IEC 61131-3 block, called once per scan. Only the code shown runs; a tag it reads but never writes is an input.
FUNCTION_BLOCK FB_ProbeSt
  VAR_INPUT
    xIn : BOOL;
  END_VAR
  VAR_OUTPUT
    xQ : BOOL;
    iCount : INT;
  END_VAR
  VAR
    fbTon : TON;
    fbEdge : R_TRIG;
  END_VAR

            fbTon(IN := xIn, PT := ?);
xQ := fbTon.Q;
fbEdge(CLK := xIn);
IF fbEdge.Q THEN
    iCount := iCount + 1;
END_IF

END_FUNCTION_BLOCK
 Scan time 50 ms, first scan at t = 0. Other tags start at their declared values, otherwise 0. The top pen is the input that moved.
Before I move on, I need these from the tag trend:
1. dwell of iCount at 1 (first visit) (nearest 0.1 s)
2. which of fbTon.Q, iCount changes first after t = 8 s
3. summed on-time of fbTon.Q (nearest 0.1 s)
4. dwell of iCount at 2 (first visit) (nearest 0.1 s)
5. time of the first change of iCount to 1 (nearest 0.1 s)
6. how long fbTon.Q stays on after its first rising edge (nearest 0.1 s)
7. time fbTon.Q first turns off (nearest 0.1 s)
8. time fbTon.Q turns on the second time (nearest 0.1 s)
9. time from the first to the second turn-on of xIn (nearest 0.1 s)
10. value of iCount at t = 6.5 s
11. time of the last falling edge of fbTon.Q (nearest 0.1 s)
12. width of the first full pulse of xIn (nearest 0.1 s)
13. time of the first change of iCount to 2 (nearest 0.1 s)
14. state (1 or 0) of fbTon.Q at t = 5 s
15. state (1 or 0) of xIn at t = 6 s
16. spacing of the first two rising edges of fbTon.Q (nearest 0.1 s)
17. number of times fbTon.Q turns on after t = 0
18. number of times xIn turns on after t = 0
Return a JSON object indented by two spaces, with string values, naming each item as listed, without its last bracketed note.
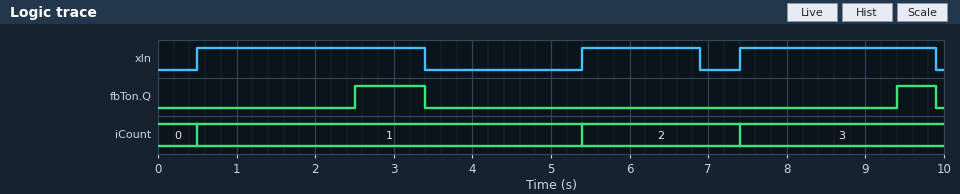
{
  "dwell of iCount at 1 (first visit)": "4.9 s",
  "which of fbTon.Q, iCount changes first after t = 8 s": "fbTon.Q",
  "summed on-time of fbTon.Q": "1.4 s",
  "dwell of iCount at 2 (first visit)": "2.0 s",
  "time of the first change of iCount to 1": "0.5 s",
  "how long fbTon.Q stays on after its first rising edge": "0.9 s",
  "time fbTon.Q first turns off": "3.4 s",
  "time fbTon.Q turns on the second time": "9.4 s",
  "time from the first to the second turn-on of xIn": "4.9 s",
  "value of iCount at t = 6.5 s": "2",
  "time of the last falling edge of fbTon.Q": "9.9 s",
  "width of the first full pulse of xIn": "2.9 s",
  "time of the first change of iCount to 2": "5.4 s",
  "state (1 or 0) of fbTon.Q at t = 5 s": "0",
  "state (1 or 0) of xIn at t = 6 s": "1",
  "spacing of the first two rising edges of fbTon.Q": "6.9 s",
  "number of times fbTon.Q turns on after t = 0": "2",
  "number of times xIn turns on after t = 0": "3"
}
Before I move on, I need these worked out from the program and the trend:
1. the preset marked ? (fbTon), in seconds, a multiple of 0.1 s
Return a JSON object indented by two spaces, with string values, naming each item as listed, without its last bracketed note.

{
  "the preset marked ? (fbTon), in seconds, a multiple of 0.1 s": "2.0 s"
}
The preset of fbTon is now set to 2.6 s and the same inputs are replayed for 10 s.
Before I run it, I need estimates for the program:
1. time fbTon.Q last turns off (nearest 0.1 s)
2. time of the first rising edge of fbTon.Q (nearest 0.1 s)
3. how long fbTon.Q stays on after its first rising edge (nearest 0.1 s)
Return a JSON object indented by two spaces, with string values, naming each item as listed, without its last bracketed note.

{
  "time fbTon.Q last turns off": "3.4 s",
  "time of the first rising edge of fbTon.Q": "3.1 s",
  "how long fbTon.Q stays on after its first rising edge": "0.3 s"
}
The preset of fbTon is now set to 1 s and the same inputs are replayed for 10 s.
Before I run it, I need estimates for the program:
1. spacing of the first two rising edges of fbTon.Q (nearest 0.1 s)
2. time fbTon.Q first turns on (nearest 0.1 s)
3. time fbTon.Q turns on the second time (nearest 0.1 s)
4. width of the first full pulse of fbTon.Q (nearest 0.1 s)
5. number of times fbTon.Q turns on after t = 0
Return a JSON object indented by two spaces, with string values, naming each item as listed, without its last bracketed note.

{
  "spacing of the first two rising edges of fbTon.Q": "4.9 s",
  "time fbTon.Q first turns on": "1.5 s",
  "time fbTon.Q turns on the second time": "6.4 s",
  "width of the first full pulse of fbTon.Q": "1.9 s",
  "number of times fbTon.Q turns on after t = 0": "3"
}
